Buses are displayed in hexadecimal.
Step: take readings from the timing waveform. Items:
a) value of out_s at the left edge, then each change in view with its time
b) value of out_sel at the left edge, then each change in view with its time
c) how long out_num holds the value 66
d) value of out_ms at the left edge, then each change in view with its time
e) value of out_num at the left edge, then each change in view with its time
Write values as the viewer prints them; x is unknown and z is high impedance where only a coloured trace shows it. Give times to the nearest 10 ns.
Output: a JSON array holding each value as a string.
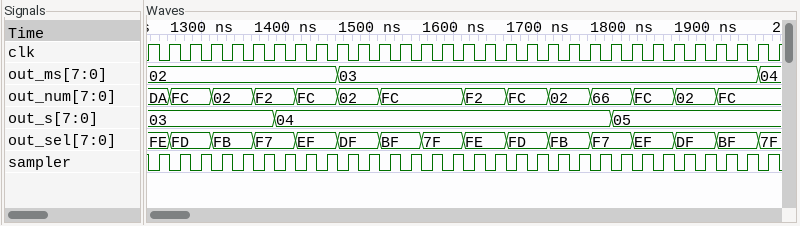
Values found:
["03, 04 at 1390 ns, 05 at 1790 ns", "FE, FD at 1260 ns, FB at 1310 ns, F7 at 1360 ns, EF at 1410 ns, DF at 1460 ns, BF at 1510 ns, 7F at 1560 ns, FE at 1610 ns, FD at 1660 ns, FB at 1710 ns, F7 at 1760 ns, EF at 1810 ns, DF at 1860 ns, BF at 1910 ns, 7F at 1960 ns", "50 ns", "02, 03 at 1460 ns, 04 at 1960 ns", "DA, FC at 1260 ns, 02 at 1310 ns, F2 at 1360 ns, FC at 1410 ns, 02 at 1460 ns, FC at 1510 ns, F2 at 1610 ns, FC at 1660 ns, 02 at 1710 ns, 66 at 1760 ns, FC at 1810 ns, 02 at 1860 ns, FC at 1910 ns"]
